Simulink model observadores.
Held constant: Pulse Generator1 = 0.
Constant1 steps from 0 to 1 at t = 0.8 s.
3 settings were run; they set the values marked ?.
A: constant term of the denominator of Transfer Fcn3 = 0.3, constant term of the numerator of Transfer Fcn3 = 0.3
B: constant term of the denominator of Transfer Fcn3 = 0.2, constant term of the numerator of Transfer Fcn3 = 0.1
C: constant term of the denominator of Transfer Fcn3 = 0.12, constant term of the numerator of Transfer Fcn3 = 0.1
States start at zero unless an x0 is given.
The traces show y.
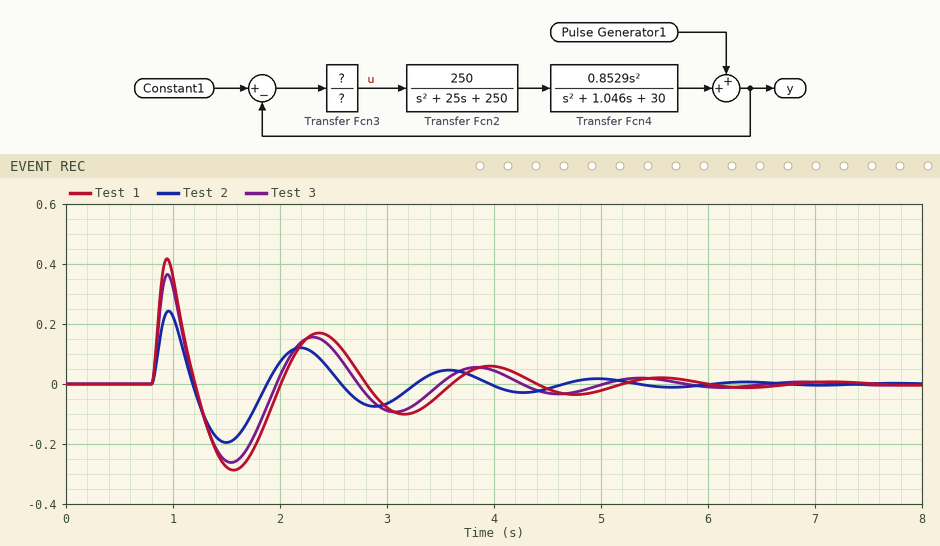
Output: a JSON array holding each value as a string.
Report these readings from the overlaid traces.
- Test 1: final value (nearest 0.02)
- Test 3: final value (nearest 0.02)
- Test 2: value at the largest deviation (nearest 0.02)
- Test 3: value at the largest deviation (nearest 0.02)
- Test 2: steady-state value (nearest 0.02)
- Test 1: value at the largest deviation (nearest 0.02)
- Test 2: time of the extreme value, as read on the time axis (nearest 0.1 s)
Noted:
["0.00", "0.00", "0.24", "0.36", "0.00", "0.42", "1.0 s"]
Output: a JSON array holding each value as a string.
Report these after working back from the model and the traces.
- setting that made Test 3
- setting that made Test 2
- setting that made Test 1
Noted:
["C", "B", "A"]
